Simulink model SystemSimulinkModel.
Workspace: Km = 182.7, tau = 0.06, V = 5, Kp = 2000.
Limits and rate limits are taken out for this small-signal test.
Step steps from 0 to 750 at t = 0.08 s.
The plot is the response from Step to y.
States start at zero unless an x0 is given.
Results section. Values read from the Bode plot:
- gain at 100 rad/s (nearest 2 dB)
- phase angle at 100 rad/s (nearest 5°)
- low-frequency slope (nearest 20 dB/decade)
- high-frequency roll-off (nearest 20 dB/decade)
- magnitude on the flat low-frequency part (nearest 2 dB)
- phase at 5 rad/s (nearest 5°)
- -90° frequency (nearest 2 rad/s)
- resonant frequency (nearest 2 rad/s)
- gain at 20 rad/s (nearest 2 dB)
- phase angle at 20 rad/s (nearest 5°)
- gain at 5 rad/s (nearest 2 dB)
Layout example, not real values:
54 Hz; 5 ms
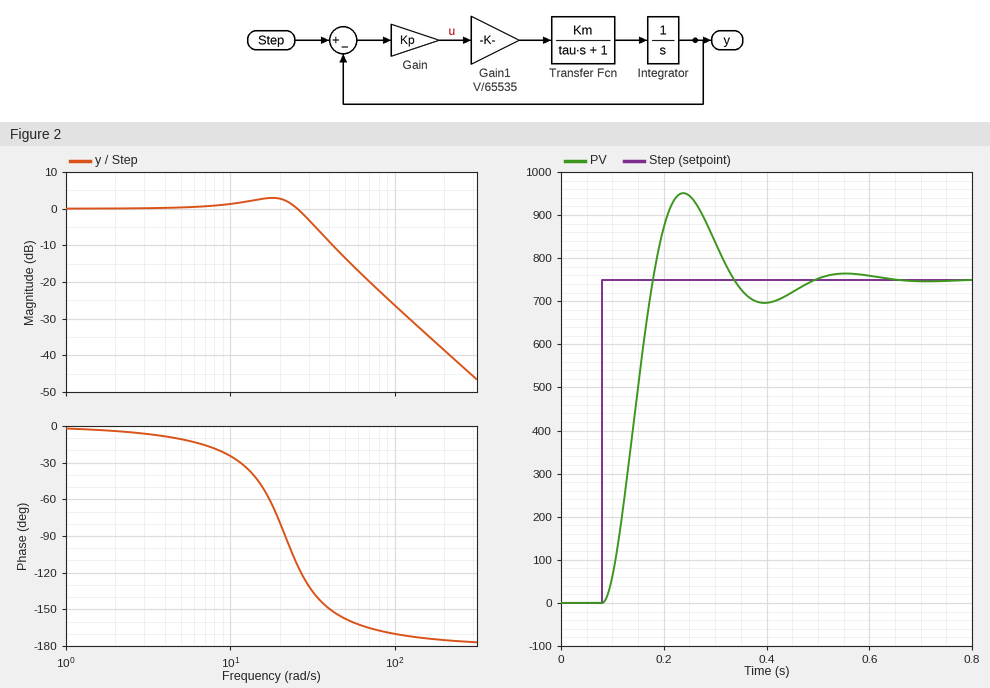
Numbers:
-26 dB; -170°; 0 dB/decade; -40 dB/decade; 0 dB; -10°; 22 rad/s; 18 rad/s; 2 dB; -80°; 0 dB
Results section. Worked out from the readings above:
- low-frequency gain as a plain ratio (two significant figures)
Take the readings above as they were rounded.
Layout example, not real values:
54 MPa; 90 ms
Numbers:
1.0
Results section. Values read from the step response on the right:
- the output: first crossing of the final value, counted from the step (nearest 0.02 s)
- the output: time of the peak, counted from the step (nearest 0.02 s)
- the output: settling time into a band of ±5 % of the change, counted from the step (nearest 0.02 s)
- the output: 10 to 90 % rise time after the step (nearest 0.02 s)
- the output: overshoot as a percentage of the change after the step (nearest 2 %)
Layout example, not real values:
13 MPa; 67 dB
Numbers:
0.10 s; 0.16 s; 0.36 s; 0.06 s; 26 %
